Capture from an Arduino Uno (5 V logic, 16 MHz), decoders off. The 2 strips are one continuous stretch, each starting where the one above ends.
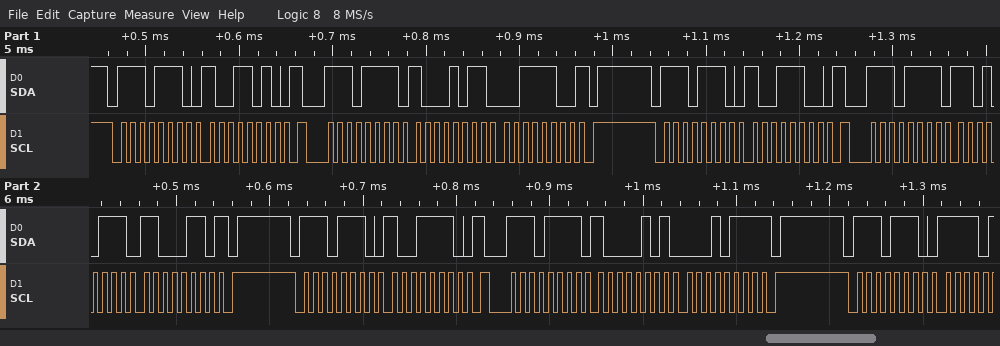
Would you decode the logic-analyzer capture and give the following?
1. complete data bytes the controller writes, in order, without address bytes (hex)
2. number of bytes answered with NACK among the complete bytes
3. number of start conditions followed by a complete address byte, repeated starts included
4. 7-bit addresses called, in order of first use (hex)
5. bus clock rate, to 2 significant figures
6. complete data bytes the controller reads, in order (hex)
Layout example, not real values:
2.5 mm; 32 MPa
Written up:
9A 9C 9E; 3; 7; 0x77; 100 kHz; 8B 3C D7 C6 85 17
